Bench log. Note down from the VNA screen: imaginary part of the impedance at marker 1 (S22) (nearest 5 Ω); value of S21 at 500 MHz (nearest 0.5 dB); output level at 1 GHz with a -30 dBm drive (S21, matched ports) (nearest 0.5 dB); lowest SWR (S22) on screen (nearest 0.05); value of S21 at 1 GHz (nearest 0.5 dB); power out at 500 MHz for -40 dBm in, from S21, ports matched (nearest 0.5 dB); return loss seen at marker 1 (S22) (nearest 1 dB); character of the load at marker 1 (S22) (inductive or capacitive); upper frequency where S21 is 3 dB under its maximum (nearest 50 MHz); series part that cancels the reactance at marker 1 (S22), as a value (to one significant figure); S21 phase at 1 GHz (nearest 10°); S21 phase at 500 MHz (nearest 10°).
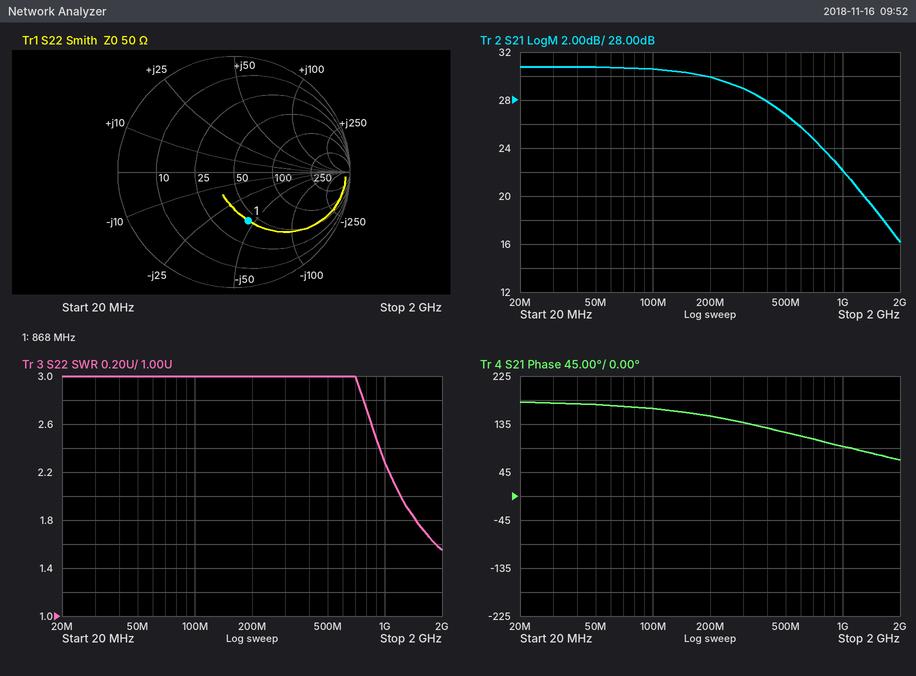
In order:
-45 Ω
27.0 dB
-8.0 dBm
1.55
22.0 dB
-13.0 dBm
7 dB
capacitive
400 MHz
8 nH
90°
120°
